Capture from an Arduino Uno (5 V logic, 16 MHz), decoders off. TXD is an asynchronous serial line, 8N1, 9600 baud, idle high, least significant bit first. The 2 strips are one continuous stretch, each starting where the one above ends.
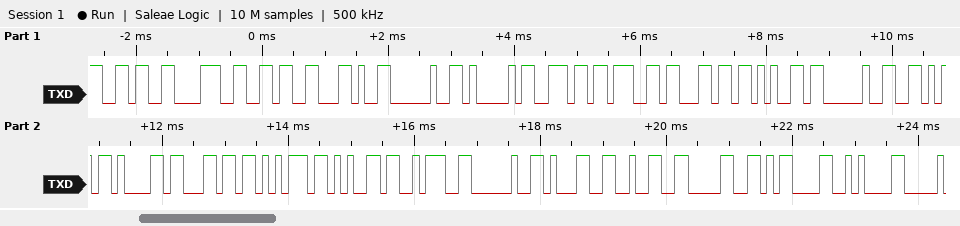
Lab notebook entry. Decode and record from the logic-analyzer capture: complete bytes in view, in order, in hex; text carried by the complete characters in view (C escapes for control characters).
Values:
36 38 36 2C 20 41 6E 67 6C 65 20 56 61 6C 75 65 3A 20 31 32 30 0D 0A
"686, Angle Value: 120\r\n"
